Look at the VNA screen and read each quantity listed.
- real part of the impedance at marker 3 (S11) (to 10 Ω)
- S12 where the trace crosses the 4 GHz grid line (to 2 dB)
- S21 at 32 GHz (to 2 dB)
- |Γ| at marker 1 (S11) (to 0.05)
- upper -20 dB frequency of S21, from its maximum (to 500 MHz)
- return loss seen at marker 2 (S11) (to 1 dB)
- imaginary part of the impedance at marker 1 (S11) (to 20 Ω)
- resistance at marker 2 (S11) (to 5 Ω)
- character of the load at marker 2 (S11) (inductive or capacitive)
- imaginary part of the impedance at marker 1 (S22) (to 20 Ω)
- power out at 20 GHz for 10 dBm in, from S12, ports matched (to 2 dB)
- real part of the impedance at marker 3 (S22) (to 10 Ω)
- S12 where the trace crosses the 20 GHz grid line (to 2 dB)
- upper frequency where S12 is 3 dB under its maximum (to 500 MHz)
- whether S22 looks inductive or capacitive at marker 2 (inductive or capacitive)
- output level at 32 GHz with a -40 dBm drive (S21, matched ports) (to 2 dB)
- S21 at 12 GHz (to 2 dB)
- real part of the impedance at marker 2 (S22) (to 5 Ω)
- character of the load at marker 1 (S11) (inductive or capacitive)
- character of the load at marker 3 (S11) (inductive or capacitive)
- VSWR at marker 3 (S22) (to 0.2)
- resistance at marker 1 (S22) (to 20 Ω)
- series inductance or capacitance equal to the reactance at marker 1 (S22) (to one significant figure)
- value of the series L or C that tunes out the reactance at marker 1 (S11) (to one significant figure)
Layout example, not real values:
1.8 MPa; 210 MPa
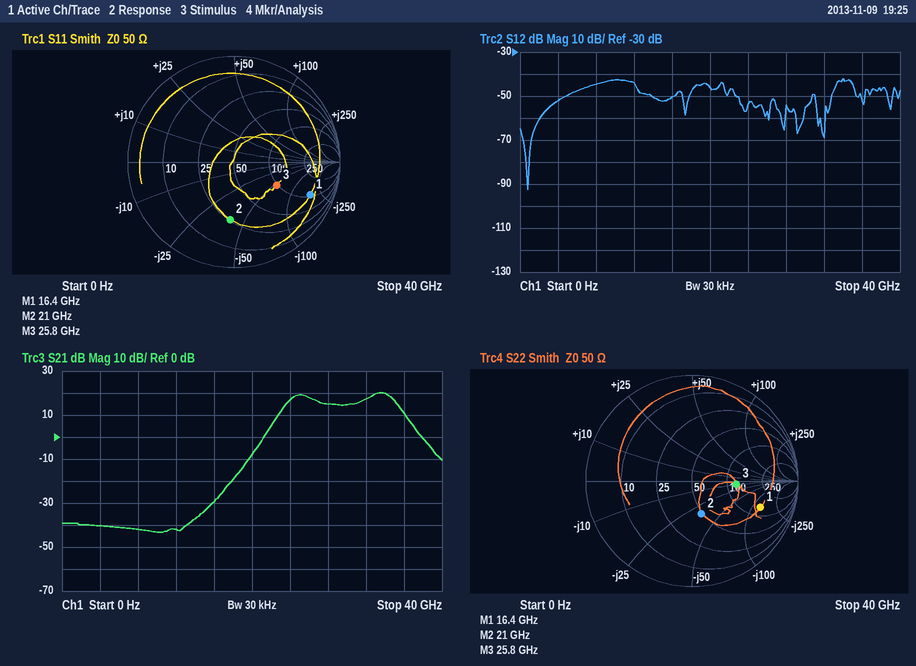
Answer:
100 Ω; -52 dB; 18 dB; 0.80; 38.0 GHz; 5 dB; -180 Ω; 25 Ω; capacitive; -140 Ω; -36 dBm; 120 Ω; -46 dB; 35.0 GHz; capacitive; -22 dBm; -42 dB; 50 Ω; capacitive; capacitive; 2.4; 140 Ω; 70 fF; 2 nH
